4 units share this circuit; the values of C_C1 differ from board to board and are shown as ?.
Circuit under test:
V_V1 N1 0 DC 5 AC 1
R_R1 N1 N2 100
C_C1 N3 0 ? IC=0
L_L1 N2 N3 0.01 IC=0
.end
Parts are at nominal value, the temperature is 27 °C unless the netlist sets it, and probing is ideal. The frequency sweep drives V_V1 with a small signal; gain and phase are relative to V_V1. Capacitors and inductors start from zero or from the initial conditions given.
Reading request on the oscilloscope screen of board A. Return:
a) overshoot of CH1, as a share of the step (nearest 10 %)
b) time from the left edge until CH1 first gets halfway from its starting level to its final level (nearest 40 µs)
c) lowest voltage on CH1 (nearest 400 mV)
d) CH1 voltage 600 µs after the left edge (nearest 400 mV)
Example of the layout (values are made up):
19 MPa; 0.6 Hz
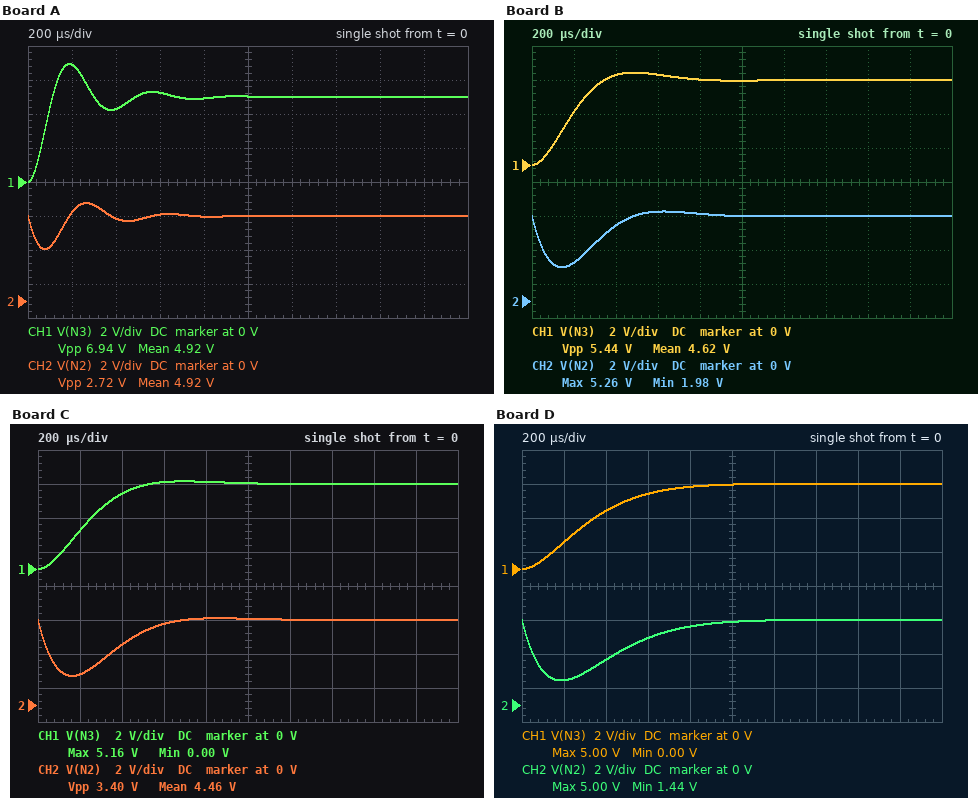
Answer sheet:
40 %; 80 µs; 0 V; 5.2 V
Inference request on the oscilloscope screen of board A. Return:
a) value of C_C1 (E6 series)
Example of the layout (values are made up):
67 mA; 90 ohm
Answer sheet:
330 nF
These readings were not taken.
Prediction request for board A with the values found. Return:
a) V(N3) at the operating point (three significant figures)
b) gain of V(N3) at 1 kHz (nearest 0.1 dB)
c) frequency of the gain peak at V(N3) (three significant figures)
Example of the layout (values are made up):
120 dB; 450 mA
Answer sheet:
5.00 V; 1.0 dB; 2.53 kHz
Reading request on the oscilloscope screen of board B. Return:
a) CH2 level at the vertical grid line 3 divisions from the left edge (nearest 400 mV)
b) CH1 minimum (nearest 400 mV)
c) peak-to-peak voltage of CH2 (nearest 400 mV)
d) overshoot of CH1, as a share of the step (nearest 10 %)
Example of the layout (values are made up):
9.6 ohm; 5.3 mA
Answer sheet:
5.2 V; 0 V; 3.2 V; 10 %
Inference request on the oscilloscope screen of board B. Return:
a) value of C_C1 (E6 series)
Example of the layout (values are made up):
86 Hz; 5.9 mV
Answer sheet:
1.5 µF
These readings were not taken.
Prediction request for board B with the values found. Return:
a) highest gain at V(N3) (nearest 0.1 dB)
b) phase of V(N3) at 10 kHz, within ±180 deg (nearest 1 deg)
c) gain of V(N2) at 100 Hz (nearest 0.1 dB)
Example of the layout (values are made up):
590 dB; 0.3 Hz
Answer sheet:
0.3 dB; -171 deg; 0 dB
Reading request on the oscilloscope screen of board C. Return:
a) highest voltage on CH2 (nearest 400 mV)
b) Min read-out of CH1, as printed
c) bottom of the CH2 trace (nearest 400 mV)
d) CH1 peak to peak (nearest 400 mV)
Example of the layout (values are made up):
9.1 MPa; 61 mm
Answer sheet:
5.2 V; 0.00 V; 1.6 V; 5.2 V
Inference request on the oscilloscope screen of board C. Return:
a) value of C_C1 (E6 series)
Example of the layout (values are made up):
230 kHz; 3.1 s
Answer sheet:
2.2 µF
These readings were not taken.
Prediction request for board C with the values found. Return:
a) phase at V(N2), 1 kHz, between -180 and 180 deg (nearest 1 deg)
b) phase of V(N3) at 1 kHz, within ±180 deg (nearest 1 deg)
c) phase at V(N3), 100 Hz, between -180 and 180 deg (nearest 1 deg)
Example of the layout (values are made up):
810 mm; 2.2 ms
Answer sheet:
-85 deg; -85 deg; -8 deg
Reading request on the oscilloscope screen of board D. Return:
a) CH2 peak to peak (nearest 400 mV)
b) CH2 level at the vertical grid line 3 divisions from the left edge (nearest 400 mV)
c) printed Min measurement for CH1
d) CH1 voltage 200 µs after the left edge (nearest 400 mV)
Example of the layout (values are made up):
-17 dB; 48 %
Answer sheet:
3.6 V; 4.0 V; 0.00 V; 1.6 V
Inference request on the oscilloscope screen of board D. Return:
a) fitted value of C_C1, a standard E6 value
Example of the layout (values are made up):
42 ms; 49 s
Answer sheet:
3.3 µF
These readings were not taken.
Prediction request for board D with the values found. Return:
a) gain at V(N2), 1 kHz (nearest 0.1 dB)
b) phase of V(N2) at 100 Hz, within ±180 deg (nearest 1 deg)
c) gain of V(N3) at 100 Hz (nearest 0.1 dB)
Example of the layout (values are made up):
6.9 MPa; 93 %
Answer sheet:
-16.8 dB; -12 deg; -0.1 dB
